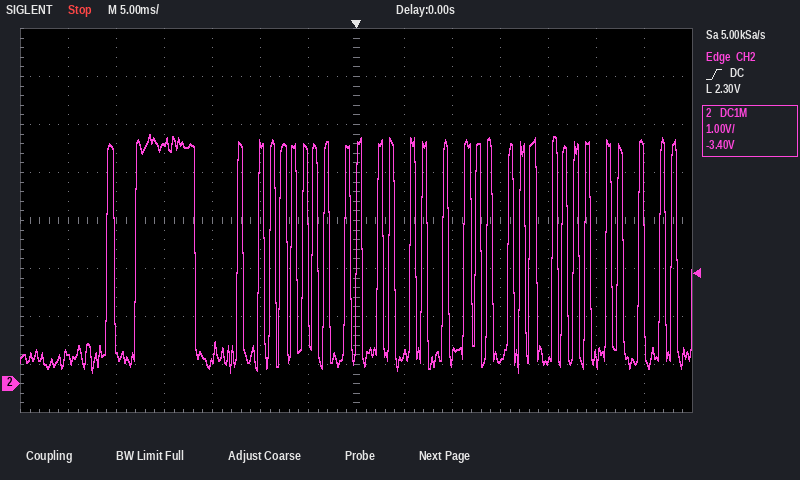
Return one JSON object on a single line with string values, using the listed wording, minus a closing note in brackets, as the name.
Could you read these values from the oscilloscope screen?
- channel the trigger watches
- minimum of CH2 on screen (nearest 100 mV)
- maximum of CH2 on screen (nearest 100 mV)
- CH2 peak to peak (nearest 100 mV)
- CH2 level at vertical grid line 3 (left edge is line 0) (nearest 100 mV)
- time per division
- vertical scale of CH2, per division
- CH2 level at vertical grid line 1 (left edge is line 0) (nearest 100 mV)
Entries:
{"channel the trigger watches": "CH2", "minimum of CH2 on screen": "200 mV", "maximum of CH2 on screen": "5.2 V", "CH2 peak to peak": "5.0 V", "CH2 level at vertical grid line 3 (left edge is line 0)": "5.0 V", "time per division": "5 ms", "vertical scale of CH2, per division": "1 V", "CH2 level at vertical grid line 1 (left edge is line 0)": "600 mV"}
